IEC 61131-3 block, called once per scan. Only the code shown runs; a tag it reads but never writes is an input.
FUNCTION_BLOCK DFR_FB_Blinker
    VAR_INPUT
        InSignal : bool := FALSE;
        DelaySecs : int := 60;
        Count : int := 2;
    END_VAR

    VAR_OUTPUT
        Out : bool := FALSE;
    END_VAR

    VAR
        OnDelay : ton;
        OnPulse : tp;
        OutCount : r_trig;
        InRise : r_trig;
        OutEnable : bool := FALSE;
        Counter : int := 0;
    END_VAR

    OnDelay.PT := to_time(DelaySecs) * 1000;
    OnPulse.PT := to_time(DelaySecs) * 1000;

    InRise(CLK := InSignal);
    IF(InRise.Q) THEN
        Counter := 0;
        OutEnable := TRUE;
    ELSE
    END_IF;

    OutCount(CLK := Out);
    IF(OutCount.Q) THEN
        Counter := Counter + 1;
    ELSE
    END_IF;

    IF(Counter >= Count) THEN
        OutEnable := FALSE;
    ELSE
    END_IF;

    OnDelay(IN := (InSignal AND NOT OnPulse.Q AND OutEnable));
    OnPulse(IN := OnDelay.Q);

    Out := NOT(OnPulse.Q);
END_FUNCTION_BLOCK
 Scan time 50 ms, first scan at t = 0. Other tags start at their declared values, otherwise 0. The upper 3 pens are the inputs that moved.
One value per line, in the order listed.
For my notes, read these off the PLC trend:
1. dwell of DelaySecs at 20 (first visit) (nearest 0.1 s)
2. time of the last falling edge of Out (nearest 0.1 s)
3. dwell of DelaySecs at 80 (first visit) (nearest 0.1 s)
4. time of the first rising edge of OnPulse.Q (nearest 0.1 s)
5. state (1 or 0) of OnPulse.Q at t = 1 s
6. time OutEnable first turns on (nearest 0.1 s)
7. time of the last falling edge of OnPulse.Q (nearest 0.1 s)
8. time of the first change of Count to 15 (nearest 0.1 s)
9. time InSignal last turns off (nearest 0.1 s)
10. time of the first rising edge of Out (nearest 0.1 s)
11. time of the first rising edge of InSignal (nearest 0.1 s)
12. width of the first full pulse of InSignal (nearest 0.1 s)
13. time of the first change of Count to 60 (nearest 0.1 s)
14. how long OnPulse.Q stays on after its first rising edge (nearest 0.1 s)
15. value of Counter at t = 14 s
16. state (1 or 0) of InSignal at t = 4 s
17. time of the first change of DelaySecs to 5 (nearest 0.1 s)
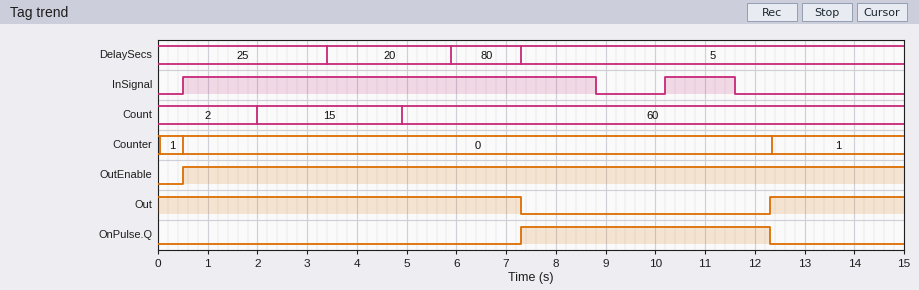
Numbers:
2.5 s
7.3 s
1.4 s
7.3 s
0
0.5 s
12.3 s
2.0 s
11.6 s
12.3 s
0.5 s
8.3 s
4.9 s
5.0 s
1
1
7.3 s
